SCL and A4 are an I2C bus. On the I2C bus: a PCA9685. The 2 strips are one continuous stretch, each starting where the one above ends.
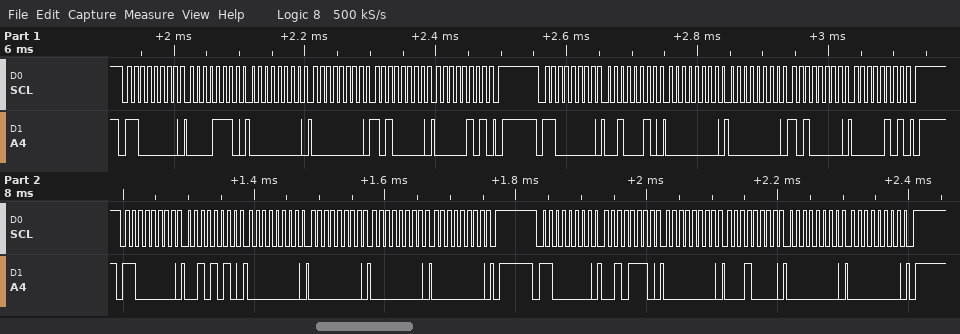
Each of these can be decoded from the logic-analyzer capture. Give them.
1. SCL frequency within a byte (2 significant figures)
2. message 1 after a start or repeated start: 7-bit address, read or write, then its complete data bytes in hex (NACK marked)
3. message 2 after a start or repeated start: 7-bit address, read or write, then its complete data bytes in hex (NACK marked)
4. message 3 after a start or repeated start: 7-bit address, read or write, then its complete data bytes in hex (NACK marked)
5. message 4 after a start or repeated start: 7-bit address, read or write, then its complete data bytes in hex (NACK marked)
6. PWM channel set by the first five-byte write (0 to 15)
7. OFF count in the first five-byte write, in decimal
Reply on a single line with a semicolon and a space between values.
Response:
100 kHz; 0x60 write: 0E 00 00 A0 05; 0x60 write: 22 00 00 A0 05; 0x60 write: 2A 00 00 00 00; 0x60 write: 2E 00 10 00 00; 2; 1440
